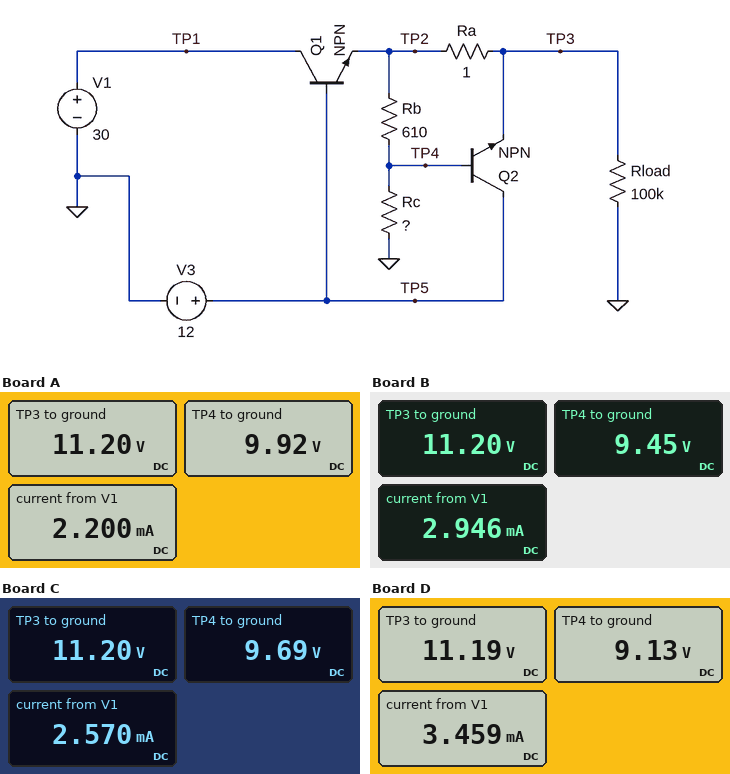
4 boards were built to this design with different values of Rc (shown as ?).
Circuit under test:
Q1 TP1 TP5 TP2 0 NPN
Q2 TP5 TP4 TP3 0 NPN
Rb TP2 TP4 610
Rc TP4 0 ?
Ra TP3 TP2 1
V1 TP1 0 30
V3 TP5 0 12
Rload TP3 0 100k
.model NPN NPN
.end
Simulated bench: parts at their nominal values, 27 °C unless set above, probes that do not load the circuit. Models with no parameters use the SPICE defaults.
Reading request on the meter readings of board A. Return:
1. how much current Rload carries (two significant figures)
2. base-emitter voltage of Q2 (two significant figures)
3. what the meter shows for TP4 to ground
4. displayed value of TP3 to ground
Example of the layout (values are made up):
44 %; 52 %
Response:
110 µA; -1.3 V; 9.92 V; 11.20 V
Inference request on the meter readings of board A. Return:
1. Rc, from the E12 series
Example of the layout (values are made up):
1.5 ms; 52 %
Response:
4.7 kΩ
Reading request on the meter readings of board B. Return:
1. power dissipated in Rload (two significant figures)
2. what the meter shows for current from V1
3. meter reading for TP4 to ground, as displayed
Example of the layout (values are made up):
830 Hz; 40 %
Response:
1.3 mW; 2.946 mA; 9.45 V
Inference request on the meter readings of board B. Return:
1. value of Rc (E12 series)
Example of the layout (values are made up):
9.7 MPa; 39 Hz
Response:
3.3 kΩ
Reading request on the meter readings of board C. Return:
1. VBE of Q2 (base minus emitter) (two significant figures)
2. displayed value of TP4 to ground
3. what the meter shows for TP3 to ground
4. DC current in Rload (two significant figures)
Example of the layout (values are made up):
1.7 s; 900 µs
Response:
-1.5 V; 9.69 V; 11.20 V; 110 µA
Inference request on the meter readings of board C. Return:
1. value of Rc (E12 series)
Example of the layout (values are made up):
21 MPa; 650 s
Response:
3.9 kΩ
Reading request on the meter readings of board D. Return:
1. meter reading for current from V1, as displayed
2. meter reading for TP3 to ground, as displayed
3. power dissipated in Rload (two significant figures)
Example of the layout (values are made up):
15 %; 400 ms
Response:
3.459 mA; 11.19 V; 1.3 mW
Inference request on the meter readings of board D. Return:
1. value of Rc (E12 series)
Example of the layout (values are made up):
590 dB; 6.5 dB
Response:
2.7 kΩ
